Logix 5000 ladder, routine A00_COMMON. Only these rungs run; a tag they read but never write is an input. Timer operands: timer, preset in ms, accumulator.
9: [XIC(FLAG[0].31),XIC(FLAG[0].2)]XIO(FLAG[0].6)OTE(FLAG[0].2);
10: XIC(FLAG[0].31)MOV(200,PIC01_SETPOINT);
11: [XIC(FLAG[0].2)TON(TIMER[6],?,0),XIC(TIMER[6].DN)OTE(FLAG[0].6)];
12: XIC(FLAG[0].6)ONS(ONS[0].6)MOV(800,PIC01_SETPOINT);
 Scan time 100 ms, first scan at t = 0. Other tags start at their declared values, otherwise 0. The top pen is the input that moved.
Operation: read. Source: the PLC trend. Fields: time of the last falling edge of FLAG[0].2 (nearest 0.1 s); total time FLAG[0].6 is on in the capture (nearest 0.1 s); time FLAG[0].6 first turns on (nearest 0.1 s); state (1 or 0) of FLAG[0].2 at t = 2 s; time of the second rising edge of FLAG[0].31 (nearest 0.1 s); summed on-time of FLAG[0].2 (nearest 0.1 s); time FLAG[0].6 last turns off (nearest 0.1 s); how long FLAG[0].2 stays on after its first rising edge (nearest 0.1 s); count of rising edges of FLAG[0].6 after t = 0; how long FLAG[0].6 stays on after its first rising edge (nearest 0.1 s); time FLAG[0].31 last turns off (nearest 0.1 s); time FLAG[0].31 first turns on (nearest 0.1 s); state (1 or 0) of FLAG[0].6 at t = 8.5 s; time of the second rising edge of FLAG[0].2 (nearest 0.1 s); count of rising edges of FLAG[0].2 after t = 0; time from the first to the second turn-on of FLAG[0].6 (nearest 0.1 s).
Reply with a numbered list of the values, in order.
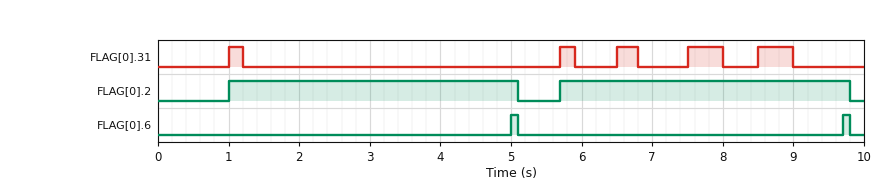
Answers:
1. 9.8 s
2. 0.2 s
3. 5.0 s
4. 1
5. 5.7 s
6. 8.2 s
7. 9.8 s
8. 4.1 s
9. 2
10. 0.1 s
11. 9.0 s
12. 1.0 s
13. 0
14. 5.7 s
15. 2
16. 4.7 s
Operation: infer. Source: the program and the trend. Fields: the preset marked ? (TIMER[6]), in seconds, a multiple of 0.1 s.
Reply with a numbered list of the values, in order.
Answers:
1. 4.0 s
